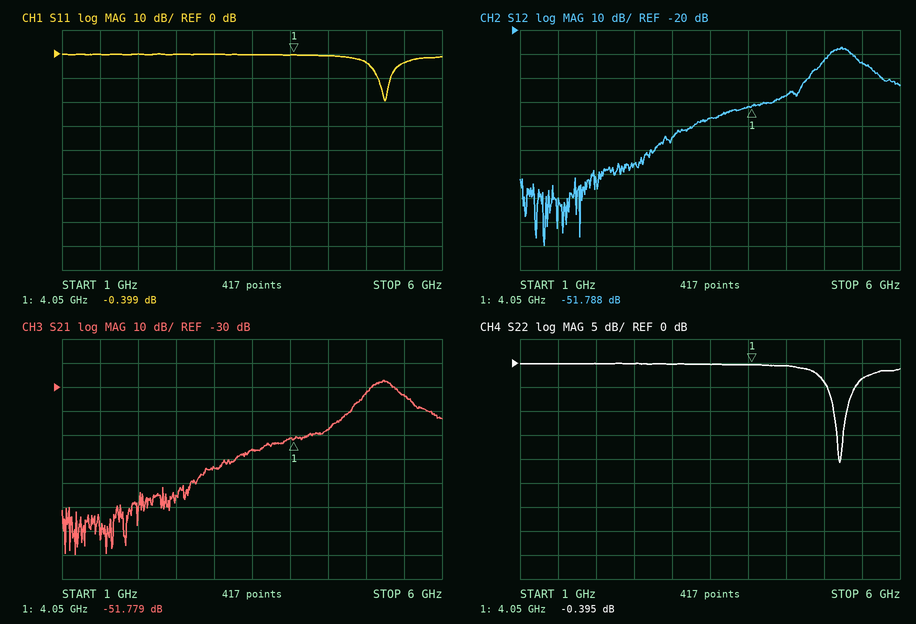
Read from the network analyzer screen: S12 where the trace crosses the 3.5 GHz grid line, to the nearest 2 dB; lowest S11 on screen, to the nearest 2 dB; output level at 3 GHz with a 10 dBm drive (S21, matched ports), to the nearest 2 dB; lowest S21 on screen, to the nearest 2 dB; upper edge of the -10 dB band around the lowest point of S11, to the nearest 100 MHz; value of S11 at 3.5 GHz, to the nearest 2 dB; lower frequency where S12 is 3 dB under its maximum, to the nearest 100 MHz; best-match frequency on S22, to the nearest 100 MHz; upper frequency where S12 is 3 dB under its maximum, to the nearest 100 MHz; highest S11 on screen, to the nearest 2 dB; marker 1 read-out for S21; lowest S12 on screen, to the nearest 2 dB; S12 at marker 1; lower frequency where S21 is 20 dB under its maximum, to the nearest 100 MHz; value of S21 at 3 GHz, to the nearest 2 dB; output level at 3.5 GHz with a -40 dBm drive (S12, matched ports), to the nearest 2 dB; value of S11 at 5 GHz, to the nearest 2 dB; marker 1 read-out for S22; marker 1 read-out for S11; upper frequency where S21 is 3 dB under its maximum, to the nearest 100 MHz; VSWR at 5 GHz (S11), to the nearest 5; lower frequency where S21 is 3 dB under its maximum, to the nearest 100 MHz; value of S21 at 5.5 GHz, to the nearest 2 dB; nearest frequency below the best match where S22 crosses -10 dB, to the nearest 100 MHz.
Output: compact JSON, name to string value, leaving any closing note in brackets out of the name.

{"S12 where the trace crosses the 3.5 GHz grid line, to the nearest 2 dB": "-56 dB", "lowest S11 on screen, to the nearest 2 dB": "-20 dB", "output level at 3 GHz with a 10 dBm drive (S21, matched ports), to the nearest 2 dB": "-54 dBm", "lowest S21 on screen, to the nearest 2 dB": "-100 dB", "upper edge of the -10 dB band around the lowest point of S11, to the nearest 100 MHz": "5.3 GHz", "value of S11 at 3.5 GHz, to the nearest 2 dB": "0 dB", "lower frequency where S12 is 3 dB under its maximum, to the nearest 100 MHz": "5.1 GHz", "best-match frequency on S22, to the nearest 100 MHz": "5.2 GHz", "upper frequency where S12 is 3 dB under its maximum, to the nearest 100 MHz": "5.4 GHz", "highest S11 on screen, to the nearest 2 dB": "0 dB", "marker 1 read-out for S21": "-51.779 dB", "lowest S12 on screen, to the nearest 2 dB": "-110 dB", "S12 at marker 1": "-51.788 dB", "lower frequency where S21 is 20 dB under its maximum, to the nearest 100 MHz": "4.5 GHz", "value of S21 at 3 GHz, to the nearest 2 dB": "-64 dB", "output level at 3.5 GHz with a -40 dBm drive (S12, matched ports), to the nearest 2 dB": "-96 dBm", "value of S11 at 5 GHz, to the nearest 2 dB": "-4 dB", "marker 1 read-out for S22": "-0.395 dB", "marker 1 read-out for S11": "-0.399 dB", "upper frequency where S21 is 3 dB under its maximum, to the nearest 100 MHz": "5.4 GHz", "VSWR at 5 GHz (S11), to the nearest 5": "5", "lower frequency where S21 is 3 dB under its maximum, to the nearest 100 MHz": "5.1 GHz", "value of S21 at 5.5 GHz, to the nearest 2 dB": "-34 dB", "nearest frequency below the best match where S22 crosses -10 dB, to the nearest 100 MHz": "5.1 GHz"}
